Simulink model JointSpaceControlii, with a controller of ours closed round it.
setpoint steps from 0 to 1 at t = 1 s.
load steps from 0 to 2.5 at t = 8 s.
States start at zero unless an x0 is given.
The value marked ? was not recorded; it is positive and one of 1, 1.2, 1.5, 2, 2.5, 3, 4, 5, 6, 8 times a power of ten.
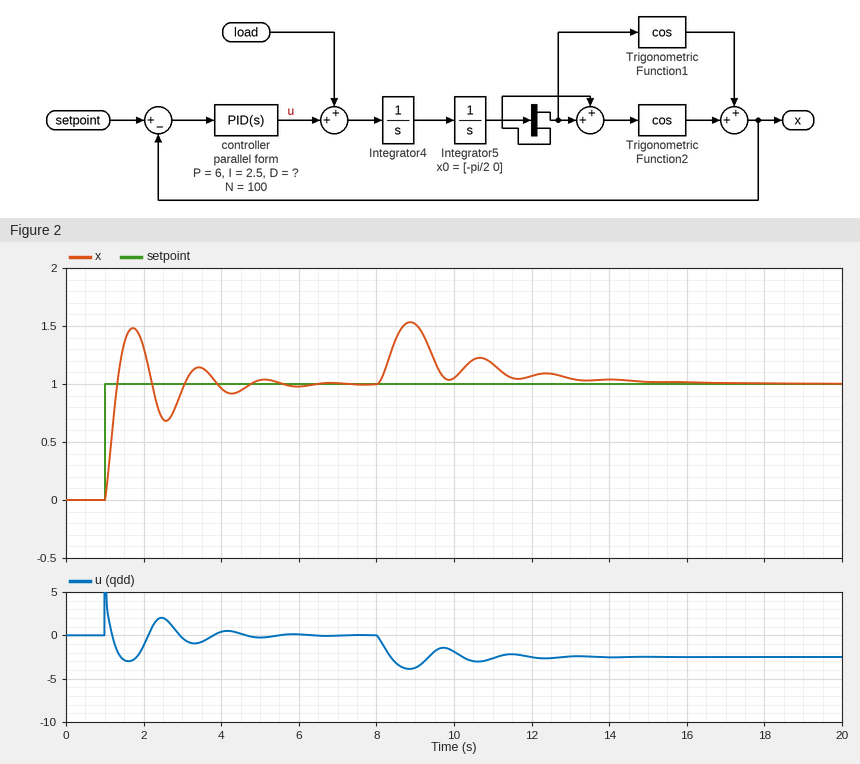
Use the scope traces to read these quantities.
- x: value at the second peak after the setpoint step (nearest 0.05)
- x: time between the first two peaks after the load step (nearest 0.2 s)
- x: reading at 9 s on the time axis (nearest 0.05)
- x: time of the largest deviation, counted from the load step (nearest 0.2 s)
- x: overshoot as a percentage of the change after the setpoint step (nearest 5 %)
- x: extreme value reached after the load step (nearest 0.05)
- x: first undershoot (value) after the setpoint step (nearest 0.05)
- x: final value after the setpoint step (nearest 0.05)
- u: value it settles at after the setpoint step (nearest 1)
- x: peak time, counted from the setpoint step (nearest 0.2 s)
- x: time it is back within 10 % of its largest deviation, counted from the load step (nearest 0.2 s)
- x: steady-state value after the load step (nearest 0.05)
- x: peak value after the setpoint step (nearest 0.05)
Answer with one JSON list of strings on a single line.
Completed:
["1.15", "1.8 s", "1.50", "0.8 s", "50 %", "1.55", "0.70", "1.00", "0", "0.8 s", "5.0 s", "1.00", "1.50"]
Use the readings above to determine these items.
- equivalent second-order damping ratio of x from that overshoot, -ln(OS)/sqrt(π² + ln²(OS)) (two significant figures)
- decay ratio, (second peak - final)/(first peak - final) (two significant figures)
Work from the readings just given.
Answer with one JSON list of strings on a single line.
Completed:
["0.22", "0.30"]
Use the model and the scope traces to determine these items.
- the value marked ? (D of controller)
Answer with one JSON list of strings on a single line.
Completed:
["0.8"]
